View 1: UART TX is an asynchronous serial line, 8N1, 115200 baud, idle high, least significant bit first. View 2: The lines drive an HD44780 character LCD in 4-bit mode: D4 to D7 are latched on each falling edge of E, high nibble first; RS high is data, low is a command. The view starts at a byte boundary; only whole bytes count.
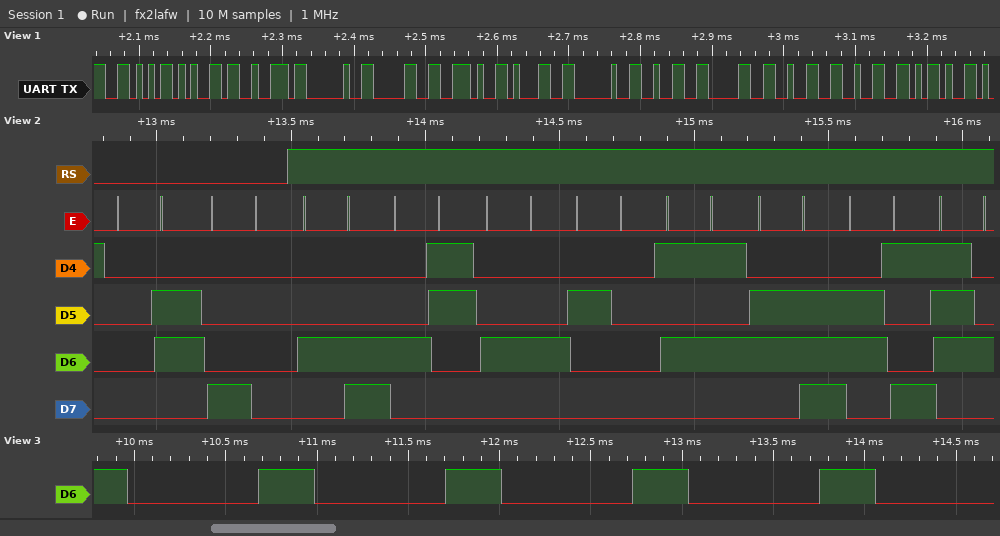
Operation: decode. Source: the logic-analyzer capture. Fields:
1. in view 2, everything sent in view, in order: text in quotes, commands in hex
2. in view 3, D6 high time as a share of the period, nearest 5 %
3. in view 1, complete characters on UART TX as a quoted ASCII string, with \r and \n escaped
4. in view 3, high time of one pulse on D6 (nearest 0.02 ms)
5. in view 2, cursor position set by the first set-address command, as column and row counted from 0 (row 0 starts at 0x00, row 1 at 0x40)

0x06 0x80 "LCD Unit"
30 %
"Ver 0.1 2022-"
0.30 ms
column 0, row 0
